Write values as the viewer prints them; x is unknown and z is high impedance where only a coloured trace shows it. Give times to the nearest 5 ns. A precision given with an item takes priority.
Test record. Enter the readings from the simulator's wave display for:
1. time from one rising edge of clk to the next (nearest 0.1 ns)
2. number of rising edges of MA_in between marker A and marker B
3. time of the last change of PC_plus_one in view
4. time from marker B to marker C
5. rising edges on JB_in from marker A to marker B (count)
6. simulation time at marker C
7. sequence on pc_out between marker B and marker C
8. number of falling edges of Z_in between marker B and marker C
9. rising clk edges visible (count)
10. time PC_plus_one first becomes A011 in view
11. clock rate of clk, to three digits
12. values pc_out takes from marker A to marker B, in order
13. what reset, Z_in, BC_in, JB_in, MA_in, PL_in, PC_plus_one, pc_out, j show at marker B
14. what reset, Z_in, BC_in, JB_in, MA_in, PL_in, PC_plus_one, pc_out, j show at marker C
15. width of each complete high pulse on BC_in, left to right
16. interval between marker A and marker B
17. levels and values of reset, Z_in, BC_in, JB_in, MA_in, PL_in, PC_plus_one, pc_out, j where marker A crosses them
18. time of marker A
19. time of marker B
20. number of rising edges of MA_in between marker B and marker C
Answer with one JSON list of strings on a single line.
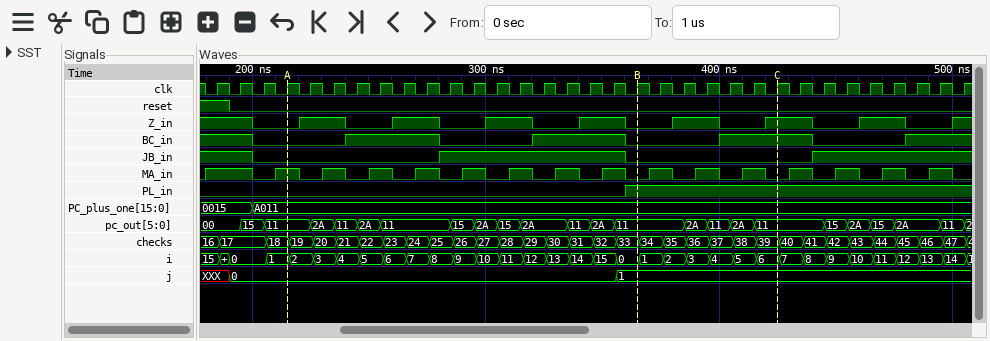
["10 ns", "7", "200 ns", "60 ns", "1", "425 ns", "11, 2A, 11, 2A, 11", "1", "33", "200 ns", "100 MHz", "11, 2A, 11, 2A, 11, 15, 2A, 15, 2A, 11, 2A, 11", "reset=0, Z_in=0, BC_in=0, JB_in=0, MA_in=0, PL_in=1, PC_plus_one=A011, pc_out=11, j=1", "reset=0, Z_in=1, BC_in=1, JB_in=0, MA_in=0, PL_in=1, PC_plus_one=A011, pc_out=11, j=1", "40 ns, 40 ns, 40 ns", "150 ns", "reset=0, Z_in=0, BC_in=0, JB_in=0, MA_in=1, PL_in=0, PC_plus_one=A011, pc_out=11, j=0", "215 ns", "365 ns", "3"]
